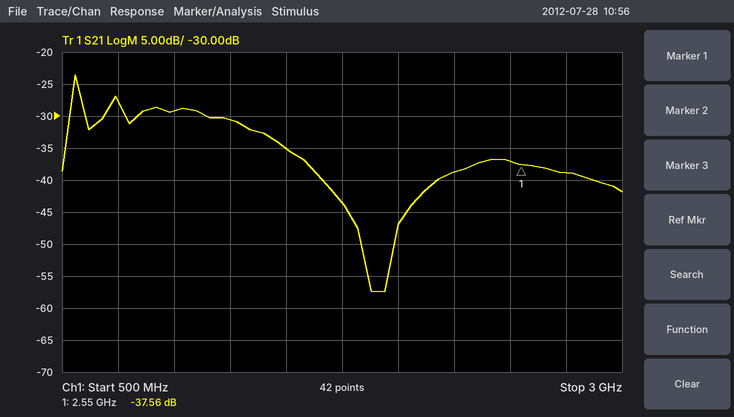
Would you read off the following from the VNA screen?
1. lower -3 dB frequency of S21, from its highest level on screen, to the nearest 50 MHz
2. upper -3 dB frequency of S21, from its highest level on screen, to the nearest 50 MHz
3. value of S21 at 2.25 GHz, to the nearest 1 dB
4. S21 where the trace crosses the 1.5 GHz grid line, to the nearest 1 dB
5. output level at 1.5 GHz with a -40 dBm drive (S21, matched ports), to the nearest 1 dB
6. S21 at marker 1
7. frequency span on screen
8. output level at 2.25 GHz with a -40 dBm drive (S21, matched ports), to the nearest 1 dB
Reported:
550 MHz
600 MHz
-39 dB
-35 dB
-75 dBm
-37.56 dB
2.5 GHz
-79 dBm
